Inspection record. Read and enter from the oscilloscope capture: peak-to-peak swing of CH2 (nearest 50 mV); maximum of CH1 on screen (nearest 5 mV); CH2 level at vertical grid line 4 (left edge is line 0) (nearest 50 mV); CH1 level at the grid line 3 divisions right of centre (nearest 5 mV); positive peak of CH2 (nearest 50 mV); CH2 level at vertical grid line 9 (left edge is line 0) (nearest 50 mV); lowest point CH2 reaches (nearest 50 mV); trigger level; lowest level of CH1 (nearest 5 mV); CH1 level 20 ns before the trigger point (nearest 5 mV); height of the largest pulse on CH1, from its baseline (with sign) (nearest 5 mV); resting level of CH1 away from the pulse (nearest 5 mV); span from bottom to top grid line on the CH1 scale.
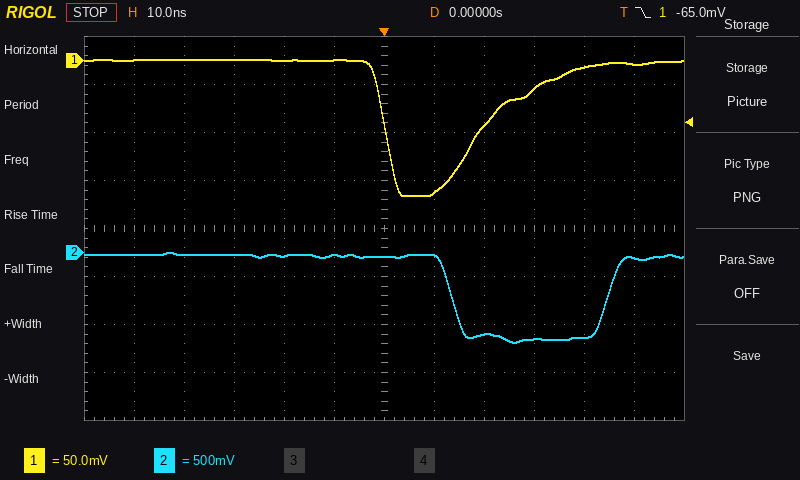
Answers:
950 mV
0 mV
-50 mV
-30 mV
0 mV
-900 mV
-950 mV
-65.0 mV
-140 mV
0 mV
-140 mV
0 mV
400 mV
